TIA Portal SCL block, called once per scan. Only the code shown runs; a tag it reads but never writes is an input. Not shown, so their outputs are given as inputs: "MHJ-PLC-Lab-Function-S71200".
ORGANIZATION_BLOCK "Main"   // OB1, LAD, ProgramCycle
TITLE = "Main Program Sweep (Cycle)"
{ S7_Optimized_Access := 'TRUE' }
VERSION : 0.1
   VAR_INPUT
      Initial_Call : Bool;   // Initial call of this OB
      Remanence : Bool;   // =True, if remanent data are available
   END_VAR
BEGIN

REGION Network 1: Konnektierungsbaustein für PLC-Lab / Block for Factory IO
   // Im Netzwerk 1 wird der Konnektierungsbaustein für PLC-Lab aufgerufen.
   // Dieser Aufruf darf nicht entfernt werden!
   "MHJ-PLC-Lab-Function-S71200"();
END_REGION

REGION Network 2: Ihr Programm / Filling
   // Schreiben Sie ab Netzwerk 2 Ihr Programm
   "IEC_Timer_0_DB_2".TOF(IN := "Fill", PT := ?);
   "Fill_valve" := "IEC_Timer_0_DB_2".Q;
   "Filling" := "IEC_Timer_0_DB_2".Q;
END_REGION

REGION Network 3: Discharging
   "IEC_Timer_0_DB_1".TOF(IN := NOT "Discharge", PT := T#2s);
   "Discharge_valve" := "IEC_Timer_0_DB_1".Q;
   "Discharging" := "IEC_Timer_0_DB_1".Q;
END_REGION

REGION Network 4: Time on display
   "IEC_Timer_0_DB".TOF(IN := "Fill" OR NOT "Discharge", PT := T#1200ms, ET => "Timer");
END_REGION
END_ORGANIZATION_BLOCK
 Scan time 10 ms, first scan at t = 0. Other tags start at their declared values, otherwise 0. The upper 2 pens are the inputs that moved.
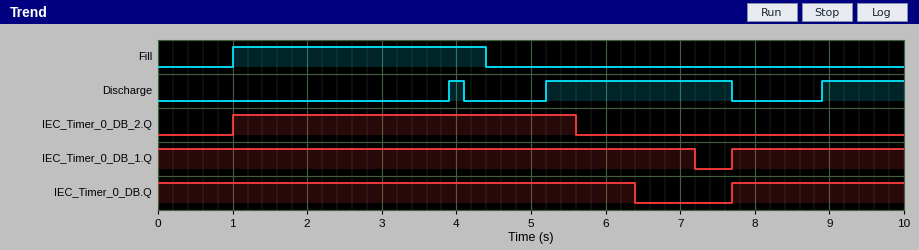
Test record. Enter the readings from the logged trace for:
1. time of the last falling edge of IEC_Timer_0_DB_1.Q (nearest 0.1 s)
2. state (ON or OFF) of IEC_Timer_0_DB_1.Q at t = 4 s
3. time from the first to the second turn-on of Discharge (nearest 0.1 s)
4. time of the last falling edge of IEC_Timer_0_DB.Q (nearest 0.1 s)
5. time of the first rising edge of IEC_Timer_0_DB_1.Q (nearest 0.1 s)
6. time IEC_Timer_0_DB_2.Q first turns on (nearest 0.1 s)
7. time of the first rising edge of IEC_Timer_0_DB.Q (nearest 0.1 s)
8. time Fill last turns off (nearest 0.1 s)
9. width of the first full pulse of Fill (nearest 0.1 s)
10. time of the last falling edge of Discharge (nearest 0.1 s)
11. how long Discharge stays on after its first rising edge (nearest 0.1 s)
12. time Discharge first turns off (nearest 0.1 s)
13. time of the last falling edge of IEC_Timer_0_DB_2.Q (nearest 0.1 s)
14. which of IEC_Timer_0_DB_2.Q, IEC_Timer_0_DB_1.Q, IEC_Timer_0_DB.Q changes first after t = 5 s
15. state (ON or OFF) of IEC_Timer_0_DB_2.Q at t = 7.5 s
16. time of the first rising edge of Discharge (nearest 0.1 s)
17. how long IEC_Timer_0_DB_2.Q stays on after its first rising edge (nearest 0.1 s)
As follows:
7.2 s
ON
1.3 s
6.4 s
7.7 s
1.0 s
7.7 s
4.4 s
3.4 s
7.7 s
0.2 s
4.1 s
5.6 s
IEC_Timer_0_DB_2.Q
OFF
3.9 s
4.6 s
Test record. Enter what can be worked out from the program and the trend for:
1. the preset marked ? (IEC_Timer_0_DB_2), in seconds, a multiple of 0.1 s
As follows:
1.2 s
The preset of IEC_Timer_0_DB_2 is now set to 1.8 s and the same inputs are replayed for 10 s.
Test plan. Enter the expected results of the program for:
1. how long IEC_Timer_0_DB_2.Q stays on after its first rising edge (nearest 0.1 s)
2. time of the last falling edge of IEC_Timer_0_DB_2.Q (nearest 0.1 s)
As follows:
5.2 s
6.2 s
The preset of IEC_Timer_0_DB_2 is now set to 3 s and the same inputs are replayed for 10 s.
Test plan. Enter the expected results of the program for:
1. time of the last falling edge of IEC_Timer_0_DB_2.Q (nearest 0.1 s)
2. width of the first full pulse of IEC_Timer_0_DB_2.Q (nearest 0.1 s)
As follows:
7.4 s
6.4 s
